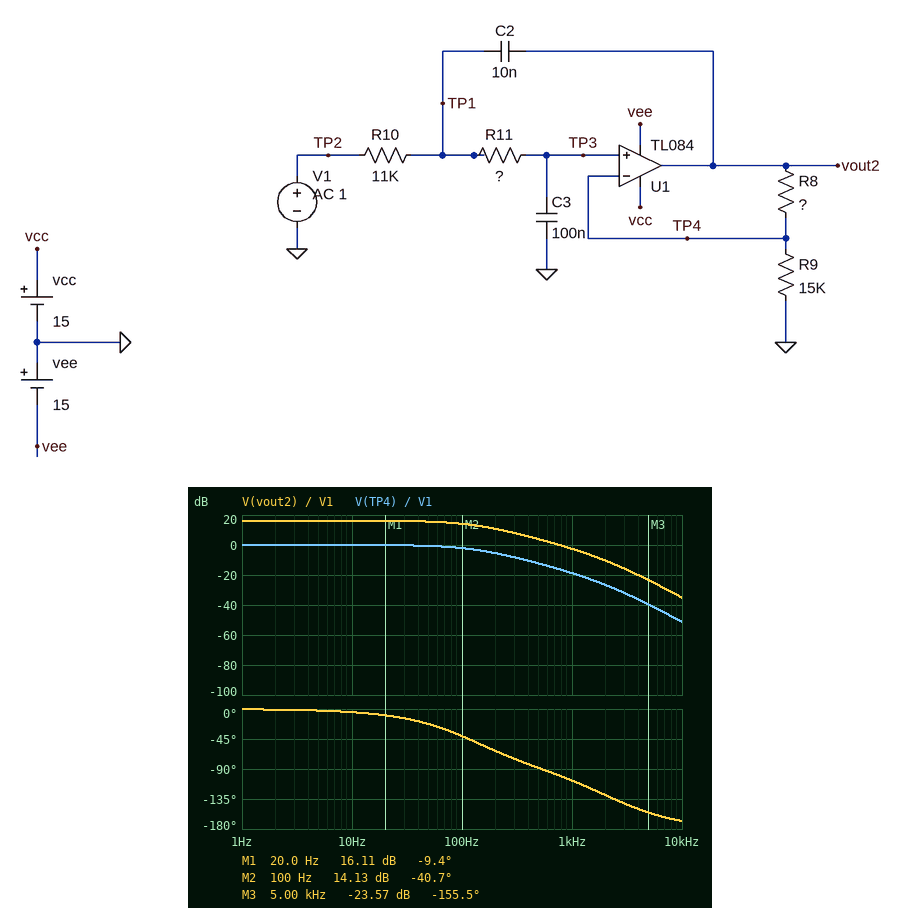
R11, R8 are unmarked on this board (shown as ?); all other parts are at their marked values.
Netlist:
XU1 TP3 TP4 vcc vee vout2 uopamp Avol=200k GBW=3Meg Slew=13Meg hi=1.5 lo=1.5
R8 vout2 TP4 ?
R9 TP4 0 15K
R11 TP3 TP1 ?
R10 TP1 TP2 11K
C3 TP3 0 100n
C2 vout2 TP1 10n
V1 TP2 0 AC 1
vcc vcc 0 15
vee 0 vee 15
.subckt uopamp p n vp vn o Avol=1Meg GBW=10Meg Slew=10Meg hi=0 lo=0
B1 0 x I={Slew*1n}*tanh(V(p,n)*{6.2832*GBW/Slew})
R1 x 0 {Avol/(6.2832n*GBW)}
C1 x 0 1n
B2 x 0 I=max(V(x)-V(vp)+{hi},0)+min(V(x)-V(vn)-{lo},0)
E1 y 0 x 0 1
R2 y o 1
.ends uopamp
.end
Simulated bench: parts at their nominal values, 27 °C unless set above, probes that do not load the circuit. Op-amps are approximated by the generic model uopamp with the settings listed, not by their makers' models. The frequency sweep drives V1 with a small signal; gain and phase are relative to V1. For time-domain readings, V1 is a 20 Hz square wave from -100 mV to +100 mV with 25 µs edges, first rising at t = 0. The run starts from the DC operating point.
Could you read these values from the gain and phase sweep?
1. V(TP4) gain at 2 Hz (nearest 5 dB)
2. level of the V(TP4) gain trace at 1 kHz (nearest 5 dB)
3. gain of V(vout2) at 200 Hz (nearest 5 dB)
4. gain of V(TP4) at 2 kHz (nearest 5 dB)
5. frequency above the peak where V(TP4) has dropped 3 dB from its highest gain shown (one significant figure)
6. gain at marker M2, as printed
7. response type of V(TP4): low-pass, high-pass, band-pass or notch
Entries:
0 dB
-20 dB
10 dB
-25 dB
100 Hz
14.13 dB
low-pass
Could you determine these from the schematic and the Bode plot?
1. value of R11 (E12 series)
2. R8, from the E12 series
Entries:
8.2 kΩ
82 kΩ
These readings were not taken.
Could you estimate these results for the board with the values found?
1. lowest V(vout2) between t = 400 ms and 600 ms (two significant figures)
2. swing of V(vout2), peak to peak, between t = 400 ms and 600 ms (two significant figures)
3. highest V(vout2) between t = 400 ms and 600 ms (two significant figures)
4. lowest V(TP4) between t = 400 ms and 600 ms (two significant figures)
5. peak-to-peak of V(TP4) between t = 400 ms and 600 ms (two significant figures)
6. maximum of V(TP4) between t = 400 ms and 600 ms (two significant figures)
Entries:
-650 mV
1.3 V
650 mV
-100 mV
200 mV
100 mV
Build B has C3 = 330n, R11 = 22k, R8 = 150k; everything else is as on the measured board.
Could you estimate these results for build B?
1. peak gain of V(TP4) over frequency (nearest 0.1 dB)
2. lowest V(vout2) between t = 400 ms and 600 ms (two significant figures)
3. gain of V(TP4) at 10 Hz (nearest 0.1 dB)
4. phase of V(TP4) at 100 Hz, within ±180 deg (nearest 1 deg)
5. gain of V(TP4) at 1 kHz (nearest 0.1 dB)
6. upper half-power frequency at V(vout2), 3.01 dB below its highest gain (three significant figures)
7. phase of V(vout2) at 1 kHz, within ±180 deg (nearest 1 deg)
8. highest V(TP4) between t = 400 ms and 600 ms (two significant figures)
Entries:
0 dB
-940 mV
-1.4 dB
-84 deg
-36.7 dB
16.4 Hz
-117 deg
86 mV
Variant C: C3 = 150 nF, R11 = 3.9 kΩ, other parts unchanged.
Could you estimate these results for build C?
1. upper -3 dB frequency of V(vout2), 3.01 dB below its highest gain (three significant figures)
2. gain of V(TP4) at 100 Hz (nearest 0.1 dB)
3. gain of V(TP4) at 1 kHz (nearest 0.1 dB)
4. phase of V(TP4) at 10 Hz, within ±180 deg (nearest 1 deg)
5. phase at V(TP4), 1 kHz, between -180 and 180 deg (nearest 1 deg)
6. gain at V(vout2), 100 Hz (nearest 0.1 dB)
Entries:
99.8 Hz
-3.0 dB
-20.3 dB
-6 deg
-99 deg
13.2 dB
